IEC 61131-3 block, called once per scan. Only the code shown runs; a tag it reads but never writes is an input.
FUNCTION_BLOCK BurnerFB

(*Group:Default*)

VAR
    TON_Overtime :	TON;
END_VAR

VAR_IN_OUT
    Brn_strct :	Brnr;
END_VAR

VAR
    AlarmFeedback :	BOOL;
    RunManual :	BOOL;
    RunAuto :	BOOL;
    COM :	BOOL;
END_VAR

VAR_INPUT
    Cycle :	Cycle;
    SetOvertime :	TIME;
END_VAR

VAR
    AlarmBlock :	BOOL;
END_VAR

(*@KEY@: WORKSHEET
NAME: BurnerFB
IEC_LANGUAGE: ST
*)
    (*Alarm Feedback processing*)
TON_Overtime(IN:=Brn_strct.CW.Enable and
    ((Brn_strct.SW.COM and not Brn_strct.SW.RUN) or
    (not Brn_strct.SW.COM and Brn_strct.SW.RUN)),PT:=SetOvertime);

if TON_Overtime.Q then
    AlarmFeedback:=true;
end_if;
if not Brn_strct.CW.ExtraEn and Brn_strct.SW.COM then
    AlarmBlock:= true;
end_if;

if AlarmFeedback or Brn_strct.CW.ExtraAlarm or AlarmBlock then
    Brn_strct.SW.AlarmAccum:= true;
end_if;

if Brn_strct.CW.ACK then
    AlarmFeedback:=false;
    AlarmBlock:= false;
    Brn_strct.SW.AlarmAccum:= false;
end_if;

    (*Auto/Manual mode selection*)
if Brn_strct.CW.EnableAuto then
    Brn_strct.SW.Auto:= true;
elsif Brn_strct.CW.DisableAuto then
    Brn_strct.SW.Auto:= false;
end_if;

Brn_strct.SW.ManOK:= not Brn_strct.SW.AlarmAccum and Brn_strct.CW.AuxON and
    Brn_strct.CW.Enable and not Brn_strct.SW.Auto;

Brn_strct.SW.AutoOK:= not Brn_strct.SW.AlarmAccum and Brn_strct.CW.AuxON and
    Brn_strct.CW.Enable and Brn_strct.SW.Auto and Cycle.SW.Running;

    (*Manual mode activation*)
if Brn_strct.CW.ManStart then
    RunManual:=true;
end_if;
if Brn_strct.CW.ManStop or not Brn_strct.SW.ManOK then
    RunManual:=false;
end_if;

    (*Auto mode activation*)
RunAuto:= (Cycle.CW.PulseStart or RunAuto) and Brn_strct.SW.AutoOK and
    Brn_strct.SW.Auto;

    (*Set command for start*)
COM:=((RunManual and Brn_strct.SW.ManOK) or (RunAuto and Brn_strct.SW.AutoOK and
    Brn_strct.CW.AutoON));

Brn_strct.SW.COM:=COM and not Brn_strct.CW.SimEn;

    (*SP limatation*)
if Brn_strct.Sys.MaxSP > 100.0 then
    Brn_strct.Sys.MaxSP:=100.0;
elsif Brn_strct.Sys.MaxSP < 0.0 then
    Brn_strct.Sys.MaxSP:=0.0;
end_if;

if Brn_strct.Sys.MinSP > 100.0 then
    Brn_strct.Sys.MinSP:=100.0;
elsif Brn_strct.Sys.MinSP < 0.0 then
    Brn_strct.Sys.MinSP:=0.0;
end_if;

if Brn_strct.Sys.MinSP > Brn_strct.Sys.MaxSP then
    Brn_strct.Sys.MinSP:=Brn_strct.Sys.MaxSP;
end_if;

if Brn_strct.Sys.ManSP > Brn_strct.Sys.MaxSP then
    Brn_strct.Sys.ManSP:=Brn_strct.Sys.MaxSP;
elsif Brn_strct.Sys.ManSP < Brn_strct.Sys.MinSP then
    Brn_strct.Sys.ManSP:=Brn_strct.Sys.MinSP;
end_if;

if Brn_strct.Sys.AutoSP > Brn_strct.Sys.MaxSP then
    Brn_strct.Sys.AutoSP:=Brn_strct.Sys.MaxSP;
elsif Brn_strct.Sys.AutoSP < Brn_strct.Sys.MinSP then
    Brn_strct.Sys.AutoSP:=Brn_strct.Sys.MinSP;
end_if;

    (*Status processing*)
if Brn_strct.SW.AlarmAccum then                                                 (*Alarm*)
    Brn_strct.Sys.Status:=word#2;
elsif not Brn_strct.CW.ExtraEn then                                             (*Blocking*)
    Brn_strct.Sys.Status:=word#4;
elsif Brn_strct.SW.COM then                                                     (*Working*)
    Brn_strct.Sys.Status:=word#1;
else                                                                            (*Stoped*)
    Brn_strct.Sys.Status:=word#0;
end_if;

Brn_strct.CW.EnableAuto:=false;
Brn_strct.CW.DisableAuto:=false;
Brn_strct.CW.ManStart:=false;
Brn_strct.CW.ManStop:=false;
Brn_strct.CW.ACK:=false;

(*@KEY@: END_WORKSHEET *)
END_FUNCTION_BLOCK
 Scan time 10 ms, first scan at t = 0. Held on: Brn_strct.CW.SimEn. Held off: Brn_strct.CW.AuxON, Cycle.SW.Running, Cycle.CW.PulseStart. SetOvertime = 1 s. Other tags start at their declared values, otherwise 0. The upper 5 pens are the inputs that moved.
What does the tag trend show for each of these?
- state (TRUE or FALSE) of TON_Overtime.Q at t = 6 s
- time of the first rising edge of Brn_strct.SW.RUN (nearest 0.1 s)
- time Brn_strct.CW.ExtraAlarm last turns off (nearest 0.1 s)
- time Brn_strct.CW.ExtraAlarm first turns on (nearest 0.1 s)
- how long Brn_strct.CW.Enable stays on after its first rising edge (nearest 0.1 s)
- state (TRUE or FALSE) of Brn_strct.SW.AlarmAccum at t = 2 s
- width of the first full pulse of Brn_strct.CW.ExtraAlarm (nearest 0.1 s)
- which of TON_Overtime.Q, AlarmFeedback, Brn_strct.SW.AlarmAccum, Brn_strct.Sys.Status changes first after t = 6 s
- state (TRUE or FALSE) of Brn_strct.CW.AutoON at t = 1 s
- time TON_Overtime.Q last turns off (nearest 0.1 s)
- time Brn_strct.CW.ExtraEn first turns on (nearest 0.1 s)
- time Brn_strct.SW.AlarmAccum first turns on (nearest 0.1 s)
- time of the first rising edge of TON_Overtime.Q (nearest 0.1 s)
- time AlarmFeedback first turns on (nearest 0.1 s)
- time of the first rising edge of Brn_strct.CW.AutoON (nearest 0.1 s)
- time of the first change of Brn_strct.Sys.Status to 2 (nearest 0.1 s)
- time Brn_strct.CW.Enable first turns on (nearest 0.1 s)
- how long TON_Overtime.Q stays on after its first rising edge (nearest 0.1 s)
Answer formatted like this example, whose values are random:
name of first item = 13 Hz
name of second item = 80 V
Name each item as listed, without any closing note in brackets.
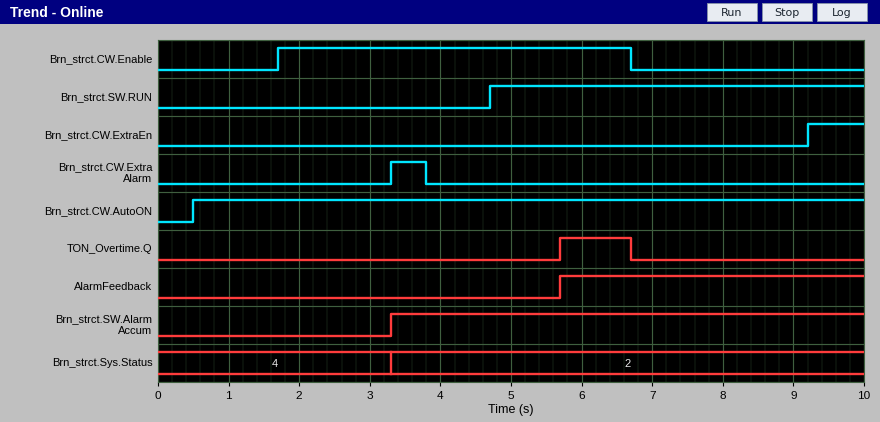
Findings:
state (TRUE or FALSE) of TON_Overtime.Q at t = 6 s = TRUE
time of the first rising edge of Brn_strct.SW.RUN = 4.7 s
time Brn_strct.CW.ExtraAlarm last turns off = 3.8 s
time Brn_strct.CW.ExtraAlarm first turns on = 3.3 s
how long Brn_strct.CW.Enable stays on after its first rising edge = 5.0 s
state (TRUE or FALSE) of Brn_strct.SW.AlarmAccum at t = 2 s = FALSE
width of the first full pulse of Brn_strct.CW.ExtraAlarm = 0.5 s
which of TON_Overtime.Q, AlarmFeedback, Brn_strct.SW.AlarmAccum, Brn_strct.Sys.Status changes first after t = 6 s = TON_Overtime.Q
state (TRUE or FALSE) of Brn_strct.CW.AutoON at t = 1 s = TRUE
time TON_Overtime.Q last turns off = 6.7 s
time Brn_strct.CW.ExtraEn first turns on = 9.2 s
time Brn_strct.SW.AlarmAccum first turns on = 3.3 s
time of the first rising edge of TON_Overtime.Q = 5.7 s
time AlarmFeedback first turns on = 5.7 s
time of the first rising edge of Brn_strct.CW.AutoON = 0.5 s
time of the first change of Brn_strct.Sys.Status to 2 = 3.3 s
time Brn_strct.CW.Enable first turns on = 1.7 s
how long TON_Overtime.Q stays on after its first rising edge = 1.0 s
